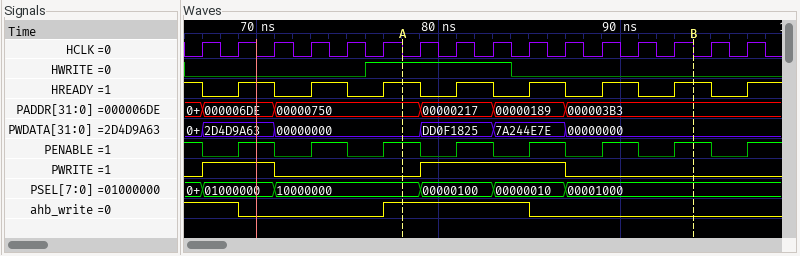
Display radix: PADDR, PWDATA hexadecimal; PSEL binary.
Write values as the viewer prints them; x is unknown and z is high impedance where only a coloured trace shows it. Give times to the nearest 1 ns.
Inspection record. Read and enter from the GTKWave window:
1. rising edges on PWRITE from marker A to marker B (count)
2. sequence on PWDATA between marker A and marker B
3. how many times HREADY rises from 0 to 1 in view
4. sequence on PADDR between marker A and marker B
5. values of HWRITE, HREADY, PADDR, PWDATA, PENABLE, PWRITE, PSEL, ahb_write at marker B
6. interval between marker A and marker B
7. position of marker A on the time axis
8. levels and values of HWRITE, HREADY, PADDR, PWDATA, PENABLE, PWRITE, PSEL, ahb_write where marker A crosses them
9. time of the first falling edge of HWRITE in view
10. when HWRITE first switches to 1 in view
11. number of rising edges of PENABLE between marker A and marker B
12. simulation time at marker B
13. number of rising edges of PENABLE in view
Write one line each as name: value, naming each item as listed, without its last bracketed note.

rising edges on PWRITE from marker A to marker B: 1
sequence on PWDATA between marker A and marker B: 00000000, DD0F1825, 7A244E7E, 00000000
how many times HREADY rises from 0 to 1 in view: 8
sequence on PADDR between marker A and marker B: 00000750, 00000217, 00000189, 000003B3
values of HWRITE, HREADY, PADDR, PWDATA, PENABLE, PWRITE, PSEL, ahb_write at marker B: HWRITE=0, HREADY=1, PADDR=000003B3, PWDATA=00000000, PENABLE=1, PWRITE=0, PSEL=00001000, ahb_write=0
interval between marker A and marker B: 16 ns
position of marker A on the time axis: 78 ns
levels and values of HWRITE, HREADY, PADDR, PWDATA, PENABLE, PWRITE, PSEL, ahb_write where marker A crosses them: HWRITE=1, HREADY=1, PADDR=00000750, PWDATA=00000000, PENABLE=1, PWRITE=0, PSEL=10000000, ahb_write=1
time of the first falling edge of HWRITE in view: 84 ns
when HWRITE first switches to 1 in view: 76 ns
number of rising edges of PENABLE between marker A and marker B: 4
simulation time at marker B: 94 ns
number of rising edges of PENABLE in view: 8
